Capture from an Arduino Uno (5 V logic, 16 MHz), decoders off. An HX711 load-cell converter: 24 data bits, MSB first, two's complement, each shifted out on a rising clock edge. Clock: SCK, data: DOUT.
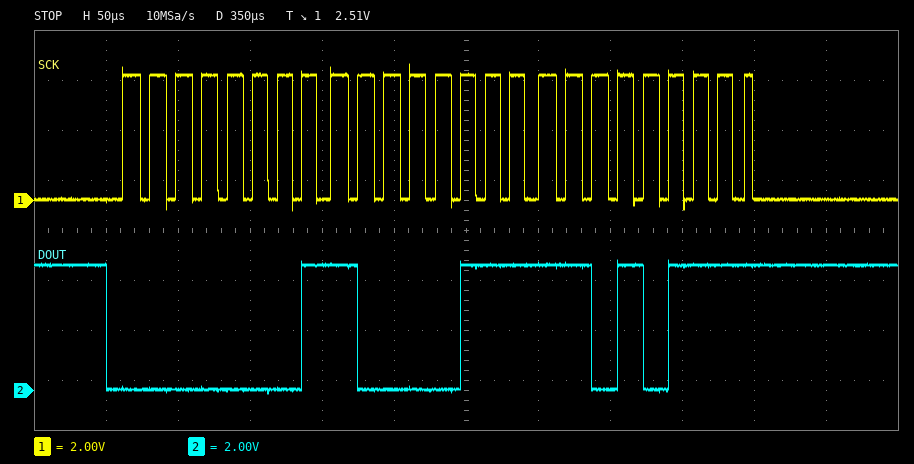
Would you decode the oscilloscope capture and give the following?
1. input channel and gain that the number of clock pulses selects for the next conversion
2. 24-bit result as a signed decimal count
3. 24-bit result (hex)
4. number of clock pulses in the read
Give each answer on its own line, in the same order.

channel A, gain 128
100311
0x0187D7
25
